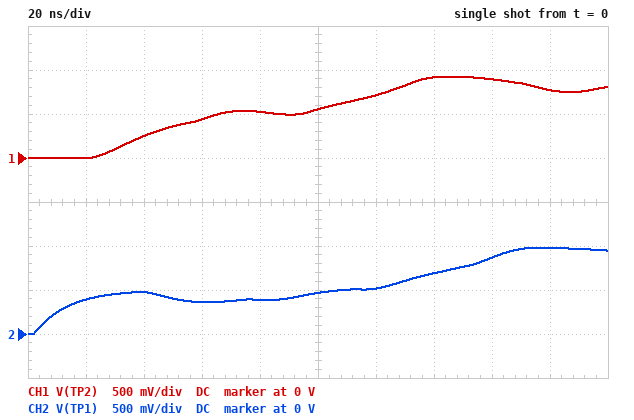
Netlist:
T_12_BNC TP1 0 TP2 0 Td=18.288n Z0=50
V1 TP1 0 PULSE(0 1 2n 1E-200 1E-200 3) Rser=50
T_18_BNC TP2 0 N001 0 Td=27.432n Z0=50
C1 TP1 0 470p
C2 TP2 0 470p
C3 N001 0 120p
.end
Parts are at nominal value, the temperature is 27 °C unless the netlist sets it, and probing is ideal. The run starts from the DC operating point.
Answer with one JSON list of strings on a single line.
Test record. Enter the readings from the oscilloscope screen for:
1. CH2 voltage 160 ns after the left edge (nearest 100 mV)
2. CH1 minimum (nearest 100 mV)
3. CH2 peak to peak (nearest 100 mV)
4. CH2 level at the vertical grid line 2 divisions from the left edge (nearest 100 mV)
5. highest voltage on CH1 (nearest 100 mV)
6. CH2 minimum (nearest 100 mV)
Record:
["900 mV", "0 V", "1.0 V", "500 mV", "900 mV", "0 V"]
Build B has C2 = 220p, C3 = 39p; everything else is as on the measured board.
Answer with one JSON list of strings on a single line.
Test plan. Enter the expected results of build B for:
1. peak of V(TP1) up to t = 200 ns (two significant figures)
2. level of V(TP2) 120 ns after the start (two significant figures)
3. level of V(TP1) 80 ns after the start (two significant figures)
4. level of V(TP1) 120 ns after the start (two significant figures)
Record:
["1.0 V", "930 mV", "450 mV", "640 mV"]
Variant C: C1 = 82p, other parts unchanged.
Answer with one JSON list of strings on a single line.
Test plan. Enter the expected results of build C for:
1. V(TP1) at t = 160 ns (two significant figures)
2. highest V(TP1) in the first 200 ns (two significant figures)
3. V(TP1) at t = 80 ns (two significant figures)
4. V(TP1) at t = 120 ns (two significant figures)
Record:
["980 mV", "1.0 V", "410 mV", "660 mV"]
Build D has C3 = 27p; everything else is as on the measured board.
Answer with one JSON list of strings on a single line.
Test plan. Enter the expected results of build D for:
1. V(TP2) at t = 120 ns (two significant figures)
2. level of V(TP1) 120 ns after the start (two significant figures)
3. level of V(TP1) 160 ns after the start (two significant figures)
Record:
["800 mV", "570 mV", "950 mV"]
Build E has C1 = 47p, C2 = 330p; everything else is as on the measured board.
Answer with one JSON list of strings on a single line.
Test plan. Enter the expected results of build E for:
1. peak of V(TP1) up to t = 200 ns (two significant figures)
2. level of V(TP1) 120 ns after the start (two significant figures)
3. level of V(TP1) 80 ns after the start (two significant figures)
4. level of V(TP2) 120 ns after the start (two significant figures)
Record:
["1.0 V", "730 mV", "500 mV", "950 mV"]
